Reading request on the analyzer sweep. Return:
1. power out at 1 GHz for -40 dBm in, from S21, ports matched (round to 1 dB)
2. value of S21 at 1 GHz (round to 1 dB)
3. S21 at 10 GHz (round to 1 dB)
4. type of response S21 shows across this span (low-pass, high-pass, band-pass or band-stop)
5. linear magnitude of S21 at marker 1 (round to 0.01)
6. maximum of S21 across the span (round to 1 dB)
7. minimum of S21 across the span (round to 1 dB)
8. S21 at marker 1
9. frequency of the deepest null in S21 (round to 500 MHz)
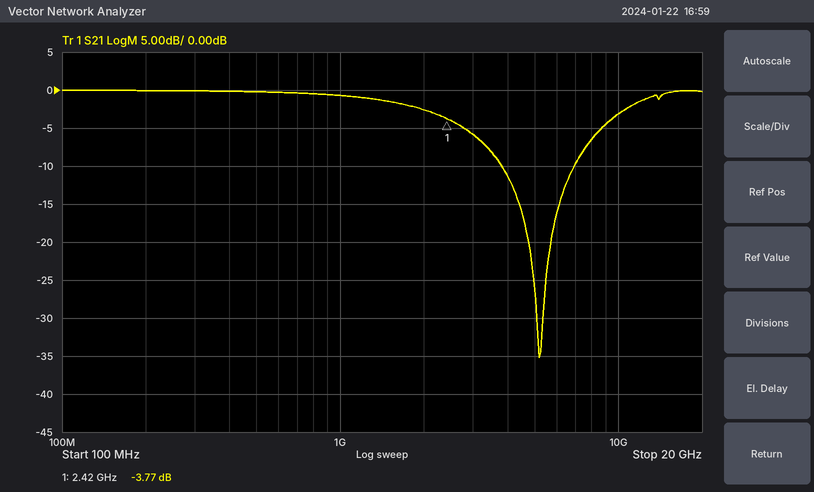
-41 dBm
-1 dB
-3 dB
band-stop
0.65
0 dB
-35 dB
-3.77 dB
5.0 GHz
